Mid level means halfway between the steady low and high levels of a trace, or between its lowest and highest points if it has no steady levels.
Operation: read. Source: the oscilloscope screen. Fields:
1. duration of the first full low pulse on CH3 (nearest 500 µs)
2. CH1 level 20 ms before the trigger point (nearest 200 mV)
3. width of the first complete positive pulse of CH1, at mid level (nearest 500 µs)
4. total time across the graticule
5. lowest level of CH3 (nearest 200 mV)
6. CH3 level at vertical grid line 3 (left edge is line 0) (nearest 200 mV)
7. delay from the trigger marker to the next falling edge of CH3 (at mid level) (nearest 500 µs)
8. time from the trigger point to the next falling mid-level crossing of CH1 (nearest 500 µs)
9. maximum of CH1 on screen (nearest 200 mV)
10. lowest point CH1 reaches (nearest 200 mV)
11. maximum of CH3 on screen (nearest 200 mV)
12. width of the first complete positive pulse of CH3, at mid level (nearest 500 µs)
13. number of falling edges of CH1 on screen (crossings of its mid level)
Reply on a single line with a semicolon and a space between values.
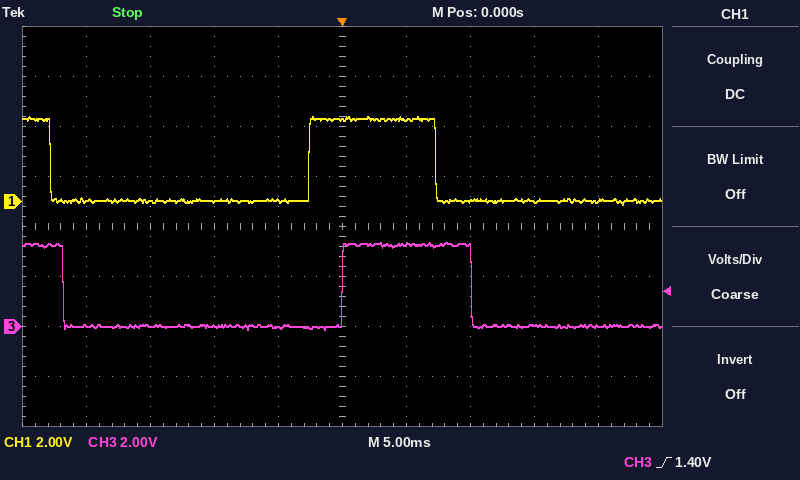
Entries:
22.0 ms; 0.0 V; 10.0 ms; 50 ms; -200 mV; 0.0 V; 10.0 ms; 7.5 ms; 3.4 V; -200 mV; 3.4 V; 10.0 ms; 2
